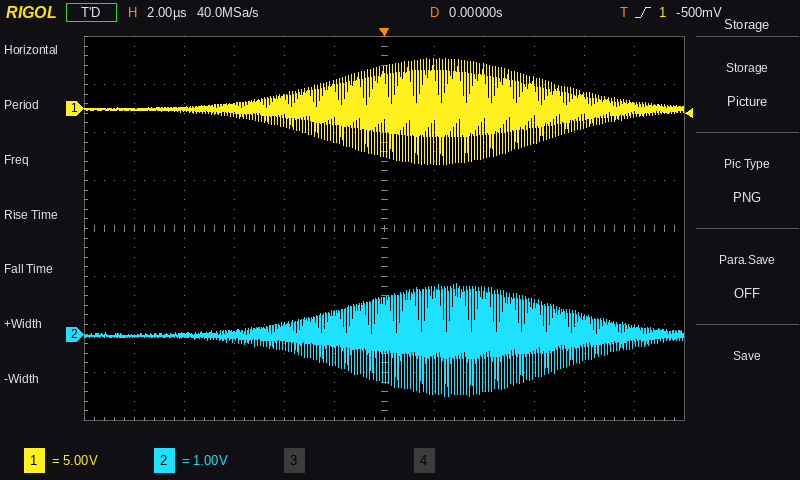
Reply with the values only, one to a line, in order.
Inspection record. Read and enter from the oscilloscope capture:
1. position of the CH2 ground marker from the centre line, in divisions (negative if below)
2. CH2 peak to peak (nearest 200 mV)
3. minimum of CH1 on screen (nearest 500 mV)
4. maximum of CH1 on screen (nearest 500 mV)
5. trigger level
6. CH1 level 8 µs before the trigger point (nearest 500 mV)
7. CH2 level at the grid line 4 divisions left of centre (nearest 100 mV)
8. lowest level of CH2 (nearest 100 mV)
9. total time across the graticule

-2.2 div
2.4 V
-5.5 V
5.0 V
-500 mV
0.0 V
0.0 V
-1.3 V
24 µs
